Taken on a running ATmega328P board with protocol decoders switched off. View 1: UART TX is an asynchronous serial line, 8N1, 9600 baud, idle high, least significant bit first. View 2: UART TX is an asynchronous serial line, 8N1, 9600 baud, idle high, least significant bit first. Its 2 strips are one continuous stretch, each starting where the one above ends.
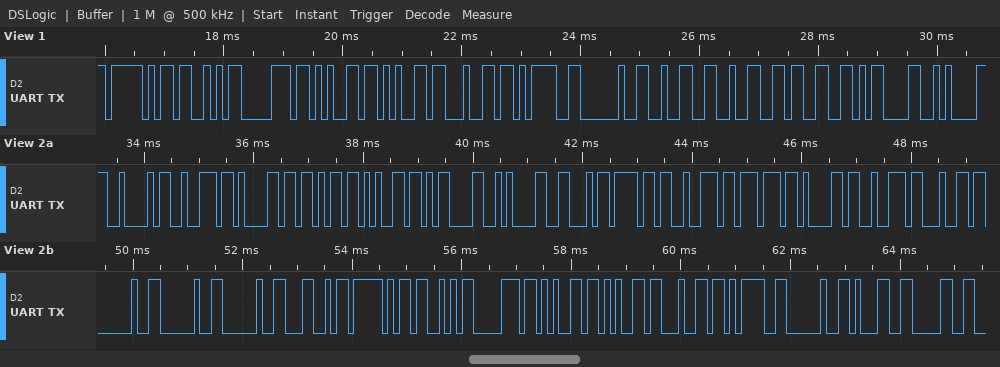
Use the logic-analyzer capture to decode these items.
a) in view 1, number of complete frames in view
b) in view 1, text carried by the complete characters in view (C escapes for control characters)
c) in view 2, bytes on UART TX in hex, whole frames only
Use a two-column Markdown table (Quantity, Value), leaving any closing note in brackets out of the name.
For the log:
| Quantity | Value |
|---|---|
| in view 1, number of complete frames in view | 13 |
| in view 1, text carried by the complete characters in view | "_Speed= 223\r\n" |
| in view 2, bytes on UART TX in hex, whole frames only | 42 72 61 6B 65 0D 0A 46 6F 72 77 61 72 64 20 20 20 4C 5F 53 70 65 65 64 3D 20 31 30 |
